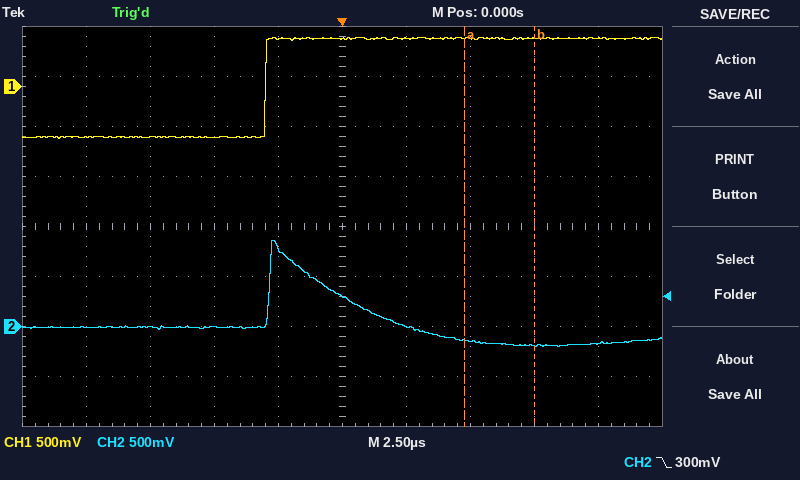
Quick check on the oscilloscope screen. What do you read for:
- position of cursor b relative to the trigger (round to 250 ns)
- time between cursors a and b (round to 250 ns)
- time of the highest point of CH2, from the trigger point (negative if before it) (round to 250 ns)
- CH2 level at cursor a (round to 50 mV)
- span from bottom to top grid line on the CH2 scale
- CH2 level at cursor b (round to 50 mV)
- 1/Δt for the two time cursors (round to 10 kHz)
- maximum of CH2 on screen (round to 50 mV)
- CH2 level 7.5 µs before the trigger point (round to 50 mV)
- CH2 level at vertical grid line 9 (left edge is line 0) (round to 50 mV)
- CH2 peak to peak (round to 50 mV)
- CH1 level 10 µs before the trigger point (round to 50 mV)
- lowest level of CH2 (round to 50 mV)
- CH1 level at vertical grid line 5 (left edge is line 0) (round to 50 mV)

+7.50 µs
2.75 µs
-2.75 µs
-150 mV
4 V
-200 mV
360 kHz
850 mV
0 mV
-150 mV
1.05 V
-500 mV
-200 mV
500 mV
